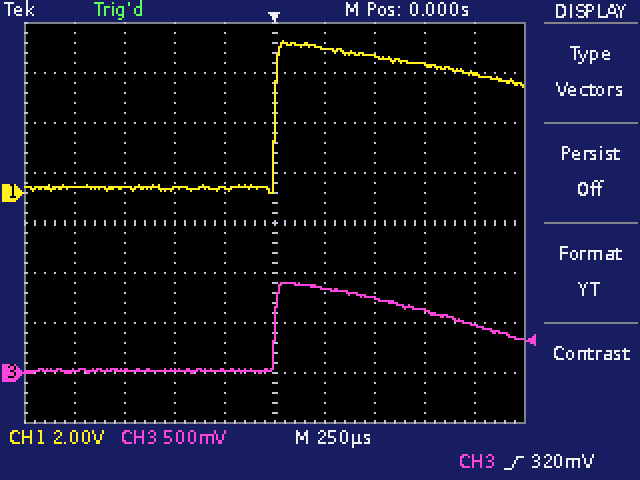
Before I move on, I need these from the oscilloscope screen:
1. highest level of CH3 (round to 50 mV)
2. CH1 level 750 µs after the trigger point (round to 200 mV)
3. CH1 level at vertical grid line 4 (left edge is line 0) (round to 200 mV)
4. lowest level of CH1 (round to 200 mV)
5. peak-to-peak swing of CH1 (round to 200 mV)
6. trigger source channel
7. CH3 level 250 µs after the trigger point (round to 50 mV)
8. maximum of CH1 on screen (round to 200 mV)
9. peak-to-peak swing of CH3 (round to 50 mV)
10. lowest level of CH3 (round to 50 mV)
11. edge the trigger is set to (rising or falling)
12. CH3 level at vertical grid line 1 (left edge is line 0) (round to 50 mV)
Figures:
900 mV
5.2 V
200 mV
0.0 V
6.0 V
CH3
850 mV
6.0 V
900 mV
0 mV
rising
0 mV
